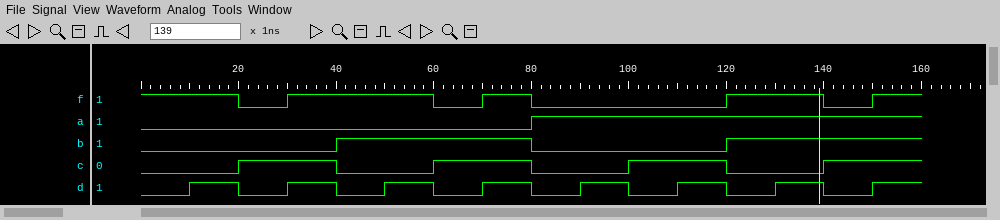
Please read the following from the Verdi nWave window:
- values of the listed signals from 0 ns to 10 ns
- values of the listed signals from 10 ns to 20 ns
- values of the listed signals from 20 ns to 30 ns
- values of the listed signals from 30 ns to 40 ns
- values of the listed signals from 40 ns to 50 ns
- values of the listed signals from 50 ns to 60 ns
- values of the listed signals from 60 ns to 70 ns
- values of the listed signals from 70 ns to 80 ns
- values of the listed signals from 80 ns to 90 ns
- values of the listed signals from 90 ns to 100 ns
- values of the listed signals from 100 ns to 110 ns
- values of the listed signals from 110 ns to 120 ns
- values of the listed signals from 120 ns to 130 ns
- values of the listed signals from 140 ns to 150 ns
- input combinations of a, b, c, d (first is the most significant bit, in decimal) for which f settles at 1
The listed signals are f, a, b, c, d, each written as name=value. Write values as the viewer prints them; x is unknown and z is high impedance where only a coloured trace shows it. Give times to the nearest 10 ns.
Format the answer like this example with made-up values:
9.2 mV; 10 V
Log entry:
f=1, a=0, b=0, c=0, d=0; f=1, a=0, b=0, c=0, d=1; f=0, a=0, b=0, c=1, d=0; f=1, a=0, b=0, c=1, d=1; f=1, a=0, b=1, c=0, d=0; f=1, a=0, b=1, c=0, d=1; f=0, a=0, b=1, c=1, d=0; f=1, a=0, b=1, c=1, d=1; f=0, a=1, b=0, c=0, d=0; f=0, a=1, b=0, c=0, d=1; f=0, a=1, b=0, c=1, d=0; f=0, a=1, b=0, c=1, d=1; f=1, a=1, b=1, c=0, d=0; f=0, a=1, b=1, c=1, d=0; 0, 1, 3, 4, 5, 7, 12, 13, 15
